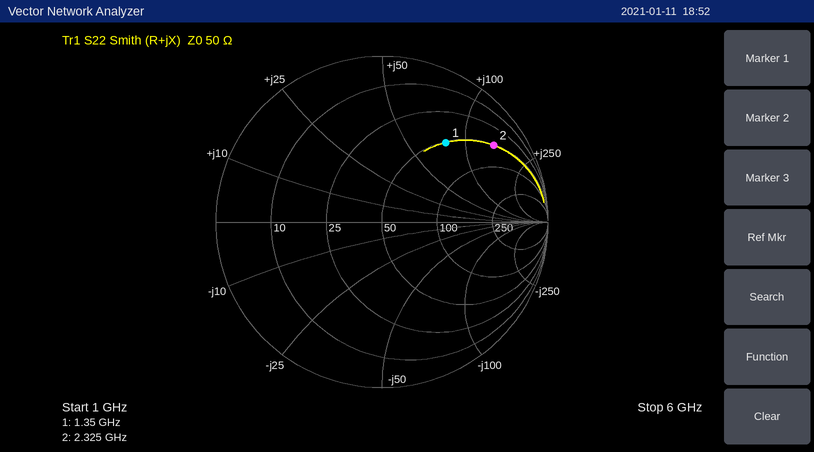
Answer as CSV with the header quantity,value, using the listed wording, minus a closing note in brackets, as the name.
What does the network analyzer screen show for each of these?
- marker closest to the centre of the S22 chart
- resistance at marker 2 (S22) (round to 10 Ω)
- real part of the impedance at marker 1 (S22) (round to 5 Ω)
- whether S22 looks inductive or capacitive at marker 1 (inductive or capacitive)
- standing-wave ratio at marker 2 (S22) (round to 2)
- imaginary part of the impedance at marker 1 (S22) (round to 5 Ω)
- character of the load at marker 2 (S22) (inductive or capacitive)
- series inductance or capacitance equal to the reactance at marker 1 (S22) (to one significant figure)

quantity,value
marker closest to the centre of the S22 chart,marker 1
resistance at marker 2 (S22),50 Ω
real part of the impedance at marker 1 (S22),50 Ω
whether S22 looks inductive or capacitive at marker 1,inductive
standing-wave ratio at marker 2 (S22),10
imaginary part of the impedance at marker 1 (S22),+80 Ω
character of the load at marker 2 (S22),inductive
series inductance or capacitance equal to the reactance at marker 1 (S22),9 nH
